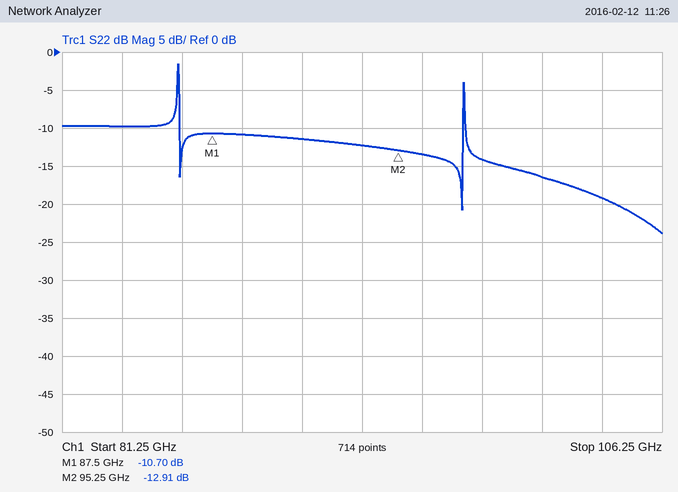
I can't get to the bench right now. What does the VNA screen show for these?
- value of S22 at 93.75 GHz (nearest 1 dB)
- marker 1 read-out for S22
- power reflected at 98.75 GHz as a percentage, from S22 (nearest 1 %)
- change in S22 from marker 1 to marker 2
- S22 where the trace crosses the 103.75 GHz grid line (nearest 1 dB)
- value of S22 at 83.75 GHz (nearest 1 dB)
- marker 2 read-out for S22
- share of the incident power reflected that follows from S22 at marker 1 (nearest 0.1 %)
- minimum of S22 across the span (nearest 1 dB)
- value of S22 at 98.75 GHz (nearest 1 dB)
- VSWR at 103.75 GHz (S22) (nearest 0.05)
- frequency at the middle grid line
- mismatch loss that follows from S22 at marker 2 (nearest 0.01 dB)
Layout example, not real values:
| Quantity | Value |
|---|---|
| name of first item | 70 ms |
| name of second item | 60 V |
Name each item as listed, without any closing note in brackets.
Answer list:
| Quantity | Value |
|---|---|
| value of S22 at 93.75 GHz | -12 dB |
| marker 1 read-out for S22 | -10.70 dB |
| power reflected at 98.75 GHz as a percentage, from S22 | 4 % |
| change in S22 from marker 1 to marker 2 | -2.21 dB |
| S22 where the trace crosses the 103.75 GHz grid line | -19 dB |
| value of S22 at 83.75 GHz | -10 dB |
| marker 2 read-out for S22 | -12.91 dB |
| share of the incident power reflected that follows from S22 at marker 1 | 8.5 % |
| minimum of S22 across the span | -24 dB |
| value of S22 at 98.75 GHz | -14 dB |
| VSWR at 103.75 GHz (S22) | 1.25 |
| frequency at the middle grid line | 93.75 GHz |
| mismatch loss that follows from S22 at marker 2 | 0.23 dB |
